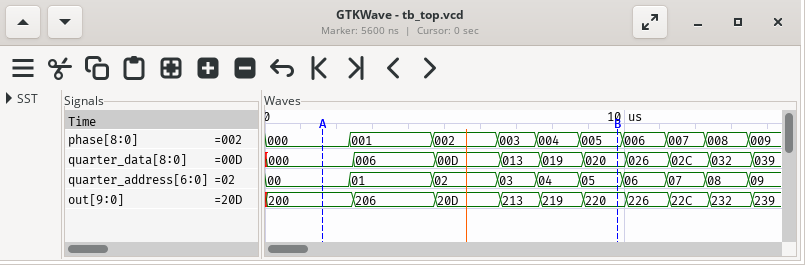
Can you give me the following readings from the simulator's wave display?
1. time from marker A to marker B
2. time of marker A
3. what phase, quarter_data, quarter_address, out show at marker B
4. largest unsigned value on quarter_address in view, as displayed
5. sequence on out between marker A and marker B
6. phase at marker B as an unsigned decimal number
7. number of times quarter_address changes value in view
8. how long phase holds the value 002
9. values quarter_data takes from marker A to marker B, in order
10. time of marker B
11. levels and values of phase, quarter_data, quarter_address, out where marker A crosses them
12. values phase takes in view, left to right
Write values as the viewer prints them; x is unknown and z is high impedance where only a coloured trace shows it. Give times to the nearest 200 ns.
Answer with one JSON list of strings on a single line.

["8200 ns", "1600 ns", "phase=005, quarter_data=020, quarter_address=05, out=220", "09", "200, 206, 20D, 213, 219, 220", "5", "9", "1800 ns", "000, 006, 00D, 013, 019, 020", "9800 ns", "phase=000, quarter_data=000, quarter_address=00, out=200", "000, 001, 002, 003, 004, 005, 006, 007, 008, 009"]
